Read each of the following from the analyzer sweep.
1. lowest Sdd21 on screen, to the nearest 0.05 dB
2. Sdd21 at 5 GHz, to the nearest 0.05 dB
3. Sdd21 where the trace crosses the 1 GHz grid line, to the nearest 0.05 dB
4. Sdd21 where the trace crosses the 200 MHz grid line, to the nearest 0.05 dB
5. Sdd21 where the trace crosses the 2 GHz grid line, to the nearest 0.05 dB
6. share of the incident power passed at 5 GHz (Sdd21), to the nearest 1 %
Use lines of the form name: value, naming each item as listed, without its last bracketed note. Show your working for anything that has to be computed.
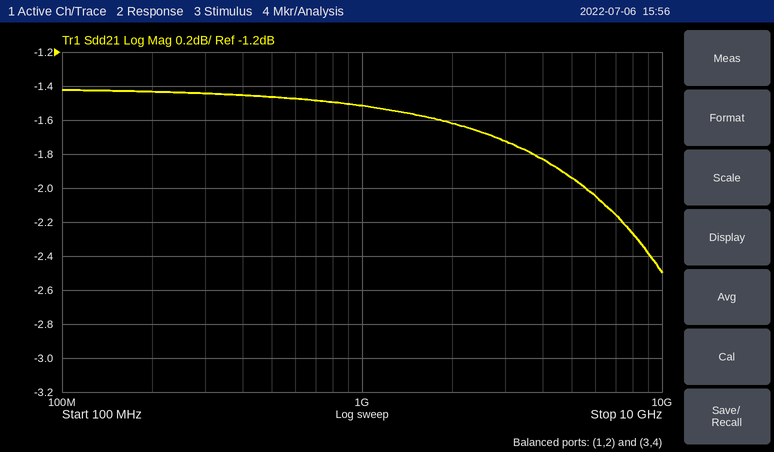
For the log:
lowest Sdd21 on screen, to the nearest 0.05 dB: -2.50 dB
Sdd21 at 5 GHz, to the nearest 0.05 dB: -1.95 dB
Sdd21 where the trace crosses the 1 GHz grid line, to the nearest 0.05 dB: -1.50 dB
Sdd21 where the trace crosses the 200 MHz grid line, to the nearest 0.05 dB: -1.45 dB
Sdd21 where the trace crosses the 2 GHz grid line, to the nearest 0.05 dB: -1.60 dB
share of the incident power passed at 5 GHz (Sdd21), to the nearest 1 %: 10^(-1.95/10) ≈ 64 %
